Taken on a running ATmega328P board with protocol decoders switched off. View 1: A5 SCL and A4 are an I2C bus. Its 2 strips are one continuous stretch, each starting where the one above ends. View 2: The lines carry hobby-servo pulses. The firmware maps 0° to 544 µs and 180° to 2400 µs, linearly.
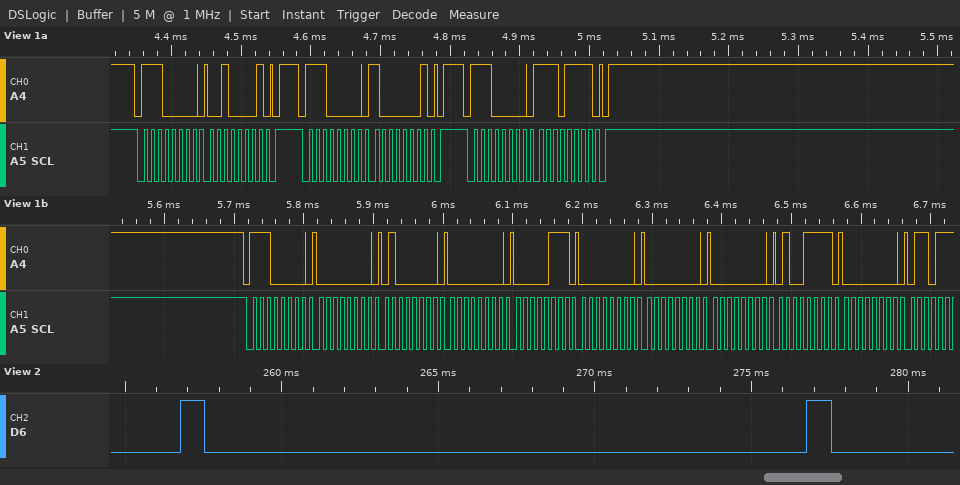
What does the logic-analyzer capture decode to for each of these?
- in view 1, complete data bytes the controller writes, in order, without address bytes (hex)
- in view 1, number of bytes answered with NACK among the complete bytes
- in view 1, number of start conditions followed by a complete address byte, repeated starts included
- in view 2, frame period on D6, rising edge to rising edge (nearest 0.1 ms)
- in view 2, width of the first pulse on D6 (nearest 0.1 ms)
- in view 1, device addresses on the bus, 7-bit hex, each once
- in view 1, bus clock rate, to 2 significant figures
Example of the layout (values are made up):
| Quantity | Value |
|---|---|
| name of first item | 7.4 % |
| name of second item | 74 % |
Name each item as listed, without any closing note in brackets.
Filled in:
| Quantity | Value |
|---|---|
| in view 1, complete data bytes the controller writes, in order, without address bytes | 21 81 EF 00 40 00 07 00 00 00 4F 00 |
| in view 1, number of bytes answered with NACK among the complete bytes | 0 |
| in view 1, number of start conditions followed by a complete address byte, repeated starts included | 4 |
| in view 2, frame period on D6, rising edge to rising edge | 20.0 ms |
| in view 2, width of the first pulse on D6 | 0.8 ms |
| in view 1, device addresses on the bus, 7-bit hex, each once | 0x70 |
| in view 1, bus clock rate, to 2 significant figures | 100 kHz |
